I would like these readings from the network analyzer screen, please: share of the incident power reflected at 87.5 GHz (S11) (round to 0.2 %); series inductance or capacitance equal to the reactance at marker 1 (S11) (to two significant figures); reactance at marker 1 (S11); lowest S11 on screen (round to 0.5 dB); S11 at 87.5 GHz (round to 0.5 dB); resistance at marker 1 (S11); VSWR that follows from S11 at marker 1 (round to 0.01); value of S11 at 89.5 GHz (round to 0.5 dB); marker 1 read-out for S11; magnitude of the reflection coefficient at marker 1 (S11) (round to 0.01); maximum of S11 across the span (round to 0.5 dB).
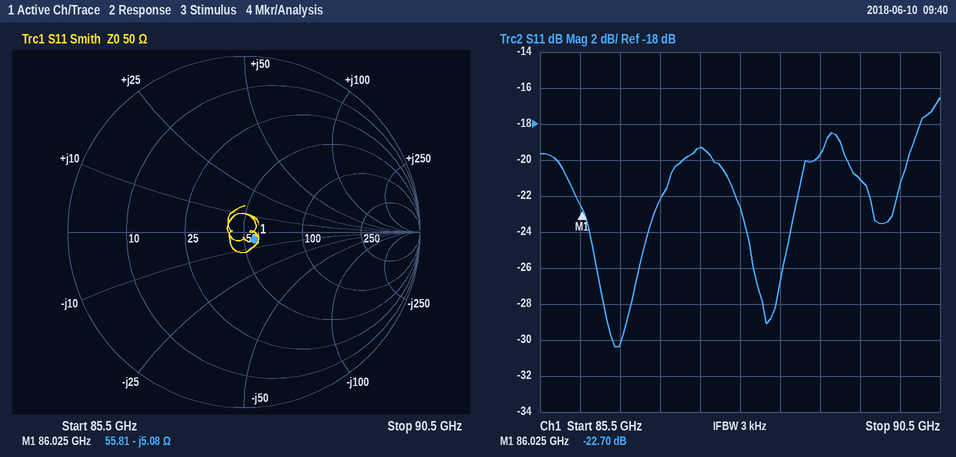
1.2 %
360 fF
-5.08 Ω
-30.5 dB
-19.5 dB
55.81 Ω
1.16
-21.0 dB
-22.70 dB
0.07
-16.5 dB
